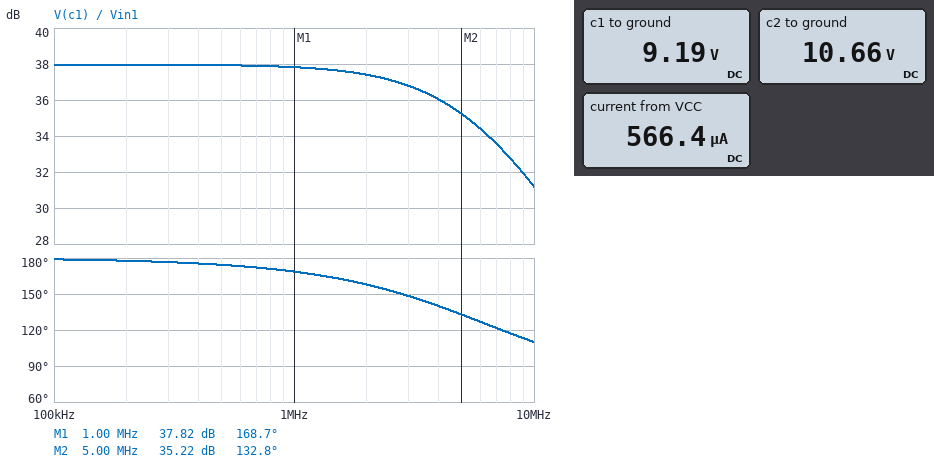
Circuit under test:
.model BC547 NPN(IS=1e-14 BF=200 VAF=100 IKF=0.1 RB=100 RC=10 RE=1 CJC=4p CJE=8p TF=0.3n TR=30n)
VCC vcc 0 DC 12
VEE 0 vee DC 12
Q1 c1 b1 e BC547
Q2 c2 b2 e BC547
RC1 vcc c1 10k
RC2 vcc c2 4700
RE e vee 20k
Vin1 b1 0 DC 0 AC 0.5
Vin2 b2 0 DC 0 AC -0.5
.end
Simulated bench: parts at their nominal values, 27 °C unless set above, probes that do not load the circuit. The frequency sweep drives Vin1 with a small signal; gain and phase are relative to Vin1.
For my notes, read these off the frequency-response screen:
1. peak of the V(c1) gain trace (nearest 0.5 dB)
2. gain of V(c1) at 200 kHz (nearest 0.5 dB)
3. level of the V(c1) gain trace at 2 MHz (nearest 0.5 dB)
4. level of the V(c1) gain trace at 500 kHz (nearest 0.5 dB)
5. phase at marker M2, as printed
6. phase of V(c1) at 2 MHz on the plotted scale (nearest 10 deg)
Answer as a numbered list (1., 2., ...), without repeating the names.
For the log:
1. 38.0 dB
2. 38.0 dB
3. 37.5 dB
4. 38.0 dB
5. 132.8 deg
6. 160 deg
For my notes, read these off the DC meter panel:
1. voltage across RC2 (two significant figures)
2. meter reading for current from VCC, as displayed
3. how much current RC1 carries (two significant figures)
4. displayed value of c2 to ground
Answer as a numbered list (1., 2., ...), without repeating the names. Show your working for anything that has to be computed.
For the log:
1. 12 V - 10.66 V = 1.3 V
2. 566.4 µA
3. (12 V - 9.19 V) / 10 kΩ = 280 µA
4. 10.66 V
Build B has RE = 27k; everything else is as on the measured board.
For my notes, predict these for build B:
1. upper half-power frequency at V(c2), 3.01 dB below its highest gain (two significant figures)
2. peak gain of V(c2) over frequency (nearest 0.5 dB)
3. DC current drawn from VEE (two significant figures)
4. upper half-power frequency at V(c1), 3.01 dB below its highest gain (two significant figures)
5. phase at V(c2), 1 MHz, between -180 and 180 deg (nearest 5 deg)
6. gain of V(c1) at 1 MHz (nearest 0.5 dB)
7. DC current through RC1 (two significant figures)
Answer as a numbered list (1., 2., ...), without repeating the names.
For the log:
1. 8.7 MHz
2. 29.0 dB
3. 420 µA
4. 6.1 MHz
5. -5 deg
6. 35.5 dB
7. 210 µA
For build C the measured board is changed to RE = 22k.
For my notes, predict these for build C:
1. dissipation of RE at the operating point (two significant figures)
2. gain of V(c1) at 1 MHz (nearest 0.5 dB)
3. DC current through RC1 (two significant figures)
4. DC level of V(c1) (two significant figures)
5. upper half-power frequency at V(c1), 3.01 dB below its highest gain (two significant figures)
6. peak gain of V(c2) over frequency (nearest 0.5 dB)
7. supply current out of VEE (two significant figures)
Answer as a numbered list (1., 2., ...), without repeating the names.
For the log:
1. 5.9 mW
2. 37.0 dB
3. 260 µA
4. 9.4 V
5. 5.6 MHz
6. 30.5 dB
7. 520 µA
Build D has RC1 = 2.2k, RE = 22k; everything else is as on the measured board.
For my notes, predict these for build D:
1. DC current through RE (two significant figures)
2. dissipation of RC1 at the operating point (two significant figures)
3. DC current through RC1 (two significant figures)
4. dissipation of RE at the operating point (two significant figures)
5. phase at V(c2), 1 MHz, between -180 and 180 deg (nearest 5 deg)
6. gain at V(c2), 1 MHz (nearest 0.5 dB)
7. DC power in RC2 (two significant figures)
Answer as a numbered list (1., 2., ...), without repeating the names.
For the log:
1. 520 µA
2. 150 µW
3. 260 µA
4. 5.9 mW
5. -5 deg
6. 30.5 dB
7. 310 µW
